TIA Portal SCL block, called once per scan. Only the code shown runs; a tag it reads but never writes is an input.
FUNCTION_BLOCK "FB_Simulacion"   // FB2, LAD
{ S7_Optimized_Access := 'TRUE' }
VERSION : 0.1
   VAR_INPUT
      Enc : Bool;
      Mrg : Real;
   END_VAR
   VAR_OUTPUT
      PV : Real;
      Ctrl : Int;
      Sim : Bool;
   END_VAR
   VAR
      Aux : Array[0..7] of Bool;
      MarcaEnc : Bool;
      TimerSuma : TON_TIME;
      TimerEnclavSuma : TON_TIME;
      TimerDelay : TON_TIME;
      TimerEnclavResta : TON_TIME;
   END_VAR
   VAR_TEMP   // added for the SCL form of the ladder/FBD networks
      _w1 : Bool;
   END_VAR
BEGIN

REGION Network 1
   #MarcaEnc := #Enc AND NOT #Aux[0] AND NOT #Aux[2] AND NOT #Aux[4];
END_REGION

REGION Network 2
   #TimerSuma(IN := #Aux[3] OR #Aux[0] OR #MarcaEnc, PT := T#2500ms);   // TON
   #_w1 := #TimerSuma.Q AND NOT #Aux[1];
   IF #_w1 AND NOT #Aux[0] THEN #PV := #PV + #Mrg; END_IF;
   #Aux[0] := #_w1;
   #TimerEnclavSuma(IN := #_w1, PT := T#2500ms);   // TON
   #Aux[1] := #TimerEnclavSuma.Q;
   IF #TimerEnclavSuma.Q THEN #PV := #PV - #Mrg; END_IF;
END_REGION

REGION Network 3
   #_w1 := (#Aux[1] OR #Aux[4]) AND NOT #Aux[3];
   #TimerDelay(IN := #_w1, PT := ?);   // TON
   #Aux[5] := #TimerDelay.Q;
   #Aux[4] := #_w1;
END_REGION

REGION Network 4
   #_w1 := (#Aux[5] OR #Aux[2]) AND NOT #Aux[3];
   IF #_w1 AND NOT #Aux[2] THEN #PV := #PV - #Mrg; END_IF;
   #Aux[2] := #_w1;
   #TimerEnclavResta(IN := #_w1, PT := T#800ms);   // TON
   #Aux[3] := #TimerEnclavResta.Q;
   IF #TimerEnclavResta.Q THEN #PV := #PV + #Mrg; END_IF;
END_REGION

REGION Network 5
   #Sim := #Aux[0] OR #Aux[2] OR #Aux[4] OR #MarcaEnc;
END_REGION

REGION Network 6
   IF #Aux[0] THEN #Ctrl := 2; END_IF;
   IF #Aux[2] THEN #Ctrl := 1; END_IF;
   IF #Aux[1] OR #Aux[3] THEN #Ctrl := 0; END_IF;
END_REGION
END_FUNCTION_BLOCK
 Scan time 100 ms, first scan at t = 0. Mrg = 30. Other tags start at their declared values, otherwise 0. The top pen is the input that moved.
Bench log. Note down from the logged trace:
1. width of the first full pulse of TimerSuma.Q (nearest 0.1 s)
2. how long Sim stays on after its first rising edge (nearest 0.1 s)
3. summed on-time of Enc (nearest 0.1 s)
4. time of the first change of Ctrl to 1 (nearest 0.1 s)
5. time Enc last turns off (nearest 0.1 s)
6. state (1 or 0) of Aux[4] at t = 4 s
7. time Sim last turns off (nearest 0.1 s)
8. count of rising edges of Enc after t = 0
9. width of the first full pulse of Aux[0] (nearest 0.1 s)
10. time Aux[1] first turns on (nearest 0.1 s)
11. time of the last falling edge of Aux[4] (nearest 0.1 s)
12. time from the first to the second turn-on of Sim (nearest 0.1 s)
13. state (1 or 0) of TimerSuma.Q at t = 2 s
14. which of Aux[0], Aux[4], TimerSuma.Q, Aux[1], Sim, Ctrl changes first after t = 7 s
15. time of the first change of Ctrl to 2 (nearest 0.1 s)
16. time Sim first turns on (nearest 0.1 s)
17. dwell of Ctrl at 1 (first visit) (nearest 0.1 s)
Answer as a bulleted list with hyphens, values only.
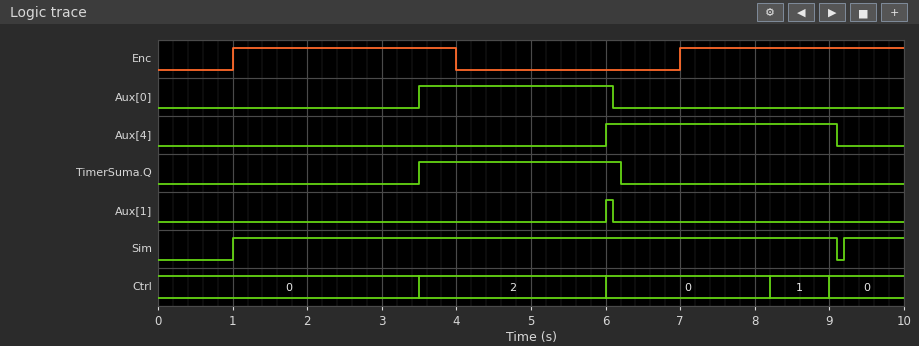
- 2.7 s
- 8.1 s
- 6.0 s
- 8.2 s
- 4.0 s
- 0
- 9.1 s
- 2
- 2.6 s
- 6.0 s
- 9.1 s
- 8.2 s
- 0
- Ctrl
- 3.5 s
- 1.0 s
- 0.8 s
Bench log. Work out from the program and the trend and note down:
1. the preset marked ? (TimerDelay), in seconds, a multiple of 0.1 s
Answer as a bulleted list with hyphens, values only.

- 2.2 s
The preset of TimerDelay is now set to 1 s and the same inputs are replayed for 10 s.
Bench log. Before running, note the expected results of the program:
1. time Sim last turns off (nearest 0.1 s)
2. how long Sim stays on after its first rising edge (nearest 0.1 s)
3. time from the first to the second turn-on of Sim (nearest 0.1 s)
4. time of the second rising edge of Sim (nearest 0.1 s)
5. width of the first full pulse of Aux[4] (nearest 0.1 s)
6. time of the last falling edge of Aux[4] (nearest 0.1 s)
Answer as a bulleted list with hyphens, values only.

- 7.9 s
- 6.9 s
- 7.0 s
- 8.0 s
- 1.9 s
- 7.9 s
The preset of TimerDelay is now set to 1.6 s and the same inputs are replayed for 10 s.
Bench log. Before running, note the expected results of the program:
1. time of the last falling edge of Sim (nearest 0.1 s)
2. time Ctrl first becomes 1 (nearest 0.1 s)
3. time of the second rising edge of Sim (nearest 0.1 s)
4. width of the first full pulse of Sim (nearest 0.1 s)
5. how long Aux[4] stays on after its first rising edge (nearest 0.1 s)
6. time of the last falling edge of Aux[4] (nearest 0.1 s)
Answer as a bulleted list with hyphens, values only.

- 8.5 s
- 7.6 s
- 8.6 s
- 7.5 s
- 2.5 s
- 8.5 s
